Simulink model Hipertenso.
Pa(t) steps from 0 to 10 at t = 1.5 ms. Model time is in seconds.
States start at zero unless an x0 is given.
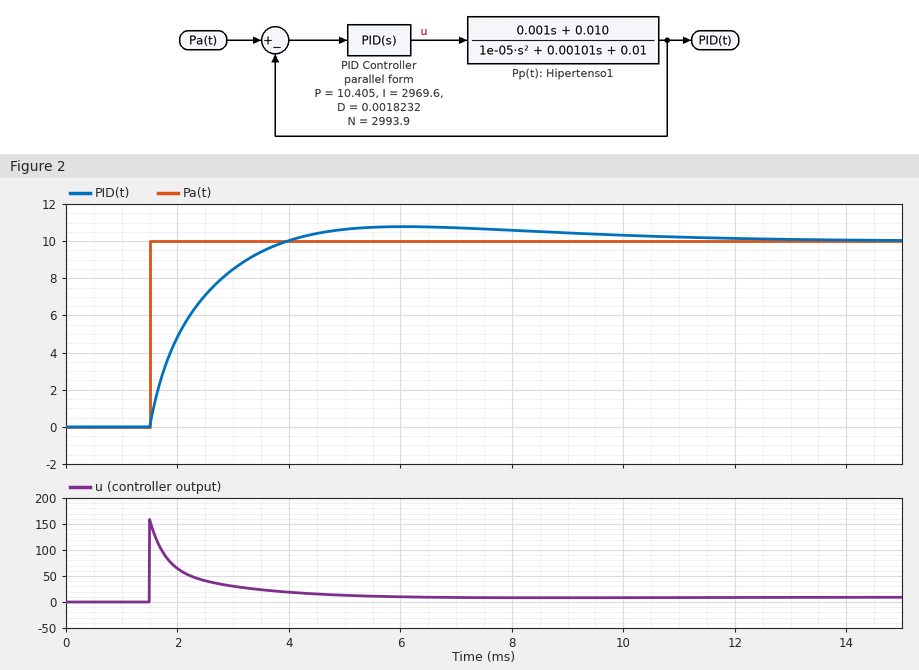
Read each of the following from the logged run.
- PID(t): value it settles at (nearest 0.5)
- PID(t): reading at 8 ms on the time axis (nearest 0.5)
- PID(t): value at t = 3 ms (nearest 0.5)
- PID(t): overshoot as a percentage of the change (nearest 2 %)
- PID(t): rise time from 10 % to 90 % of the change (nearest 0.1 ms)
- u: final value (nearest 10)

10.0
10.5
8.5
8 %
1.7 ms
10
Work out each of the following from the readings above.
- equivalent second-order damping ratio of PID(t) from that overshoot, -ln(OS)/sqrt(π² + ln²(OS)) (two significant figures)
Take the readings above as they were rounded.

0.63
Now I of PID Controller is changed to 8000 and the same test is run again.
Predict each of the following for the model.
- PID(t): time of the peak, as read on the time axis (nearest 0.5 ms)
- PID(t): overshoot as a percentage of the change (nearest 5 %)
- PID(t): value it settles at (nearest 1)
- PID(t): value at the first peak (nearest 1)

4.5 ms
20 %
10
12
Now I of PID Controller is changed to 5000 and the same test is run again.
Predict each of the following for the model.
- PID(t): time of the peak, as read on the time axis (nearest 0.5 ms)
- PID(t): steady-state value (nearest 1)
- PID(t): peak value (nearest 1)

5.0 ms
10
11
